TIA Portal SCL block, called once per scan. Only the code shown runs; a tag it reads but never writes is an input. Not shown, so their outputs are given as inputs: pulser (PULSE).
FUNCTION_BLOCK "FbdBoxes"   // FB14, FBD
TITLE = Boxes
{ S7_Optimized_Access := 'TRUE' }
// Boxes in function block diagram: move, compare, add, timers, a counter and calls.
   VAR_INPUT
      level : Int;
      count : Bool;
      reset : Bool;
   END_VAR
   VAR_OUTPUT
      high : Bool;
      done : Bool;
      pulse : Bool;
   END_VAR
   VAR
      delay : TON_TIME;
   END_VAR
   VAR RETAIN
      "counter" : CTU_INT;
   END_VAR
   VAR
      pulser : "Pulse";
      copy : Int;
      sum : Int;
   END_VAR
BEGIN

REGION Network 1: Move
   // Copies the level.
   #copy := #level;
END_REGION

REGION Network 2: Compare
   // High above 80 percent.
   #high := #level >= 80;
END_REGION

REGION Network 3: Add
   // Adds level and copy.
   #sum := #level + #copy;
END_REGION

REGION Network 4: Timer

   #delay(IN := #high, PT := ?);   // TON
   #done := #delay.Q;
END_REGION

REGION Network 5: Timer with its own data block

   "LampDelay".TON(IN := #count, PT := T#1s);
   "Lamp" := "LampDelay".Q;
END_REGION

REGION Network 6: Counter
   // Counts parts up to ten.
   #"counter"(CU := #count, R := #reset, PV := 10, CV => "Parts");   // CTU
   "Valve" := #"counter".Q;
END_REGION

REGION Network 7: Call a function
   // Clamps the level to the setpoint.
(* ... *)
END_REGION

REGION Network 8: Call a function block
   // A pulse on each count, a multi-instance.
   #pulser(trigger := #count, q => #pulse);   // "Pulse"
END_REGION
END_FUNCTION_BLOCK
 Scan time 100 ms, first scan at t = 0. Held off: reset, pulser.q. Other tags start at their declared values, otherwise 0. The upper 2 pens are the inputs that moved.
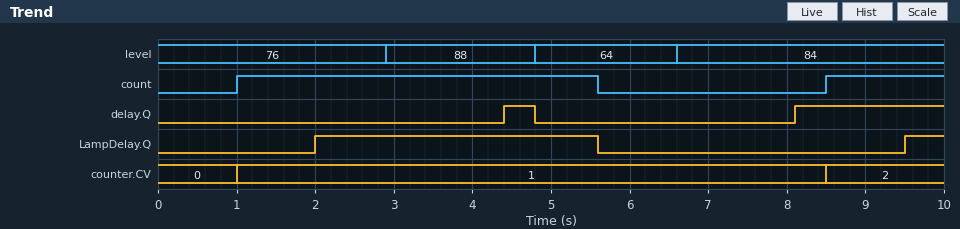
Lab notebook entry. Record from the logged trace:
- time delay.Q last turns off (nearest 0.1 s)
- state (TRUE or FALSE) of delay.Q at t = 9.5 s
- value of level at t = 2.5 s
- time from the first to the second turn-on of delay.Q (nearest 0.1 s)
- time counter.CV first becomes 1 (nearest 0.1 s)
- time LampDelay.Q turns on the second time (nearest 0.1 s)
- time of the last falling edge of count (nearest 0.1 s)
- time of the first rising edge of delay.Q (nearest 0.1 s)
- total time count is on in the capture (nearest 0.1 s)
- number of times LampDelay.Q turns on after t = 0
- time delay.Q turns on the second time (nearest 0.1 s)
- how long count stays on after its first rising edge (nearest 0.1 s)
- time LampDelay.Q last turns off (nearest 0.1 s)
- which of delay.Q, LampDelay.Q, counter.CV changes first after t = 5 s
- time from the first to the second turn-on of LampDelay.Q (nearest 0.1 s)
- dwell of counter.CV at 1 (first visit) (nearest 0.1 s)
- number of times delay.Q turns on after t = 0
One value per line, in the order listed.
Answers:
4.8 s
TRUE
76
3.7 s
1.0 s
9.5 s
5.6 s
4.4 s
6.1 s
2
8.1 s
4.6 s
5.6 s
LampDelay.Q
7.5 s
7.5 s
2
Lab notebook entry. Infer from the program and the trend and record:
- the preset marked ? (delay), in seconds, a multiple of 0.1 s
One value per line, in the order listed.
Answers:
1.5 s
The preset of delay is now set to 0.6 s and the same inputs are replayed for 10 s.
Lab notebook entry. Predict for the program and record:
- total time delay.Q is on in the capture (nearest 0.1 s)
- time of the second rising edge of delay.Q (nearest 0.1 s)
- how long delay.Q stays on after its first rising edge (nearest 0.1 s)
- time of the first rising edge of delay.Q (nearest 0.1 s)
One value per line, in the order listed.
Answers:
4.1 s
7.2 s
1.3 s
3.5 s
